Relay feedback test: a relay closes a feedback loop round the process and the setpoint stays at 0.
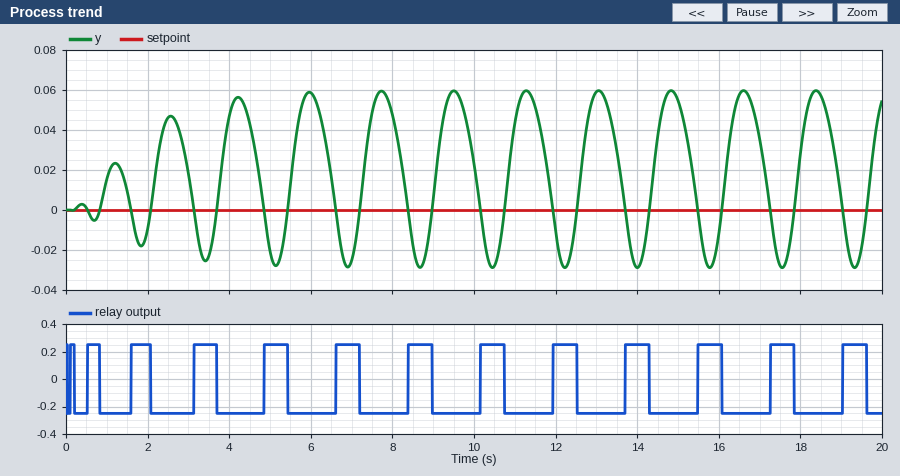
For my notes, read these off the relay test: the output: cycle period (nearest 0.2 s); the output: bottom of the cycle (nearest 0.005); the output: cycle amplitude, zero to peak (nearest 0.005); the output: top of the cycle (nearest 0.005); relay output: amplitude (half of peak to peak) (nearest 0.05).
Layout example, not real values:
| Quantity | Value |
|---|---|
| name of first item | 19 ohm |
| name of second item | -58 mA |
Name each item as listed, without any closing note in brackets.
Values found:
| Quantity | Value |
|---|---|
| the output: cycle period | 1.8 s |
| the output: bottom of the cycle | -0.030 |
| the output: cycle amplitude, zero to peak | 0.045 |
| the output: top of the cycle | 0.060 |
| relay output: amplitude (half of peak to peak) | 0.25 |
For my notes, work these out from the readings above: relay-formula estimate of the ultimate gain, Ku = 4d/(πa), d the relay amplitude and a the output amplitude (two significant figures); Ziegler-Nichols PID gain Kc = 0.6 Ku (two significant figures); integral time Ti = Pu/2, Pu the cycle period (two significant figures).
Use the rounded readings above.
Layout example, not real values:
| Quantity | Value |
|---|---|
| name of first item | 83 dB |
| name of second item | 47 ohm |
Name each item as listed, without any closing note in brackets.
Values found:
| Quantity | Value |
|---|---|
| relay-formula estimate of the ultimate gain, Ku = 4d/(πa), d the relay amplitude and a the output amplitude | 7.1 |
| Ziegler-Nichols PID gain Kc = 0.6 Ku | 4.3 |
| integral time Ti = Pu/2, Pu the cycle period | 0.90 s |
